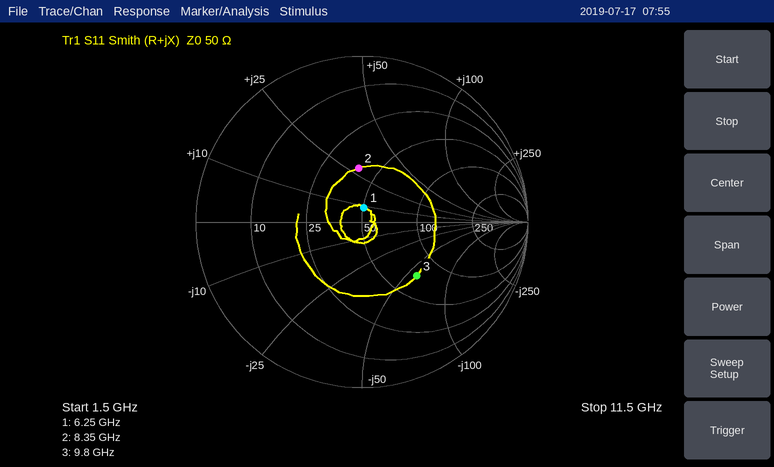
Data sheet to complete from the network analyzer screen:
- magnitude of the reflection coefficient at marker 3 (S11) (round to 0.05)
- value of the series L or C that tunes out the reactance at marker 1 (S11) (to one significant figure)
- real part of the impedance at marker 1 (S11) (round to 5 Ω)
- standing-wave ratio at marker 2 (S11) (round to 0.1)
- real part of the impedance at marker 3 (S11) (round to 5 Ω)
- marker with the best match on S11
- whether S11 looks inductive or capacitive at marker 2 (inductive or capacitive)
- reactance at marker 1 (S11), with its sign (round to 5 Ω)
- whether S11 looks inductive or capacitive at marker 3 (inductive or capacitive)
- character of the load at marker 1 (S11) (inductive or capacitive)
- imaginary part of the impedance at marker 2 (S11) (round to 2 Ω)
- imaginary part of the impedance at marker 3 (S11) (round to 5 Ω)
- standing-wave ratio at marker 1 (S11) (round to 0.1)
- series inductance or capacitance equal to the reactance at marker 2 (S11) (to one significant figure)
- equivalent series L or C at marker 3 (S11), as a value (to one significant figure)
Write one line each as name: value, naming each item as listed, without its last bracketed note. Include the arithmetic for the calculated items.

magnitude of the reflection coefficient at marker 3 (S11): 0.45
value of the series L or C that tunes out the reactance at marker 1 (S11): C = 1/(2π × 6.25 GHz × 10 Ω) ≈ 3 pF
real part of the impedance at marker 1 (S11): 50 Ω
standing-wave ratio at marker 2 (S11): 2.0
real part of the impedance at marker 3 (S11): 70 Ω
marker with the best match on S11: marker 1
whether S11 looks inductive or capacitive at marker 2: inductive
reactance at marker 1 (S11), with its sign: +10 Ω
whether S11 looks inductive or capacitive at marker 3: capacitive
character of the load at marker 1 (S11): inductive
imaginary part of the impedance at marker 2 (S11): +28 Ω
imaginary part of the impedance at marker 3 (S11): -60 Ω
standing-wave ratio at marker 1 (S11): 1.2
series inductance or capacitance equal to the reactance at marker 2 (S11): L = 28 Ω/(2π × 8.35 GHz) ≈ 534 pH, so 500 pH to one significant figure
equivalent series L or C at marker 3 (S11), as a value: C = 1/(2π × 9.8 GHz × 60 Ω) ≈ 271 fF, so 300 fF to one significant figure
